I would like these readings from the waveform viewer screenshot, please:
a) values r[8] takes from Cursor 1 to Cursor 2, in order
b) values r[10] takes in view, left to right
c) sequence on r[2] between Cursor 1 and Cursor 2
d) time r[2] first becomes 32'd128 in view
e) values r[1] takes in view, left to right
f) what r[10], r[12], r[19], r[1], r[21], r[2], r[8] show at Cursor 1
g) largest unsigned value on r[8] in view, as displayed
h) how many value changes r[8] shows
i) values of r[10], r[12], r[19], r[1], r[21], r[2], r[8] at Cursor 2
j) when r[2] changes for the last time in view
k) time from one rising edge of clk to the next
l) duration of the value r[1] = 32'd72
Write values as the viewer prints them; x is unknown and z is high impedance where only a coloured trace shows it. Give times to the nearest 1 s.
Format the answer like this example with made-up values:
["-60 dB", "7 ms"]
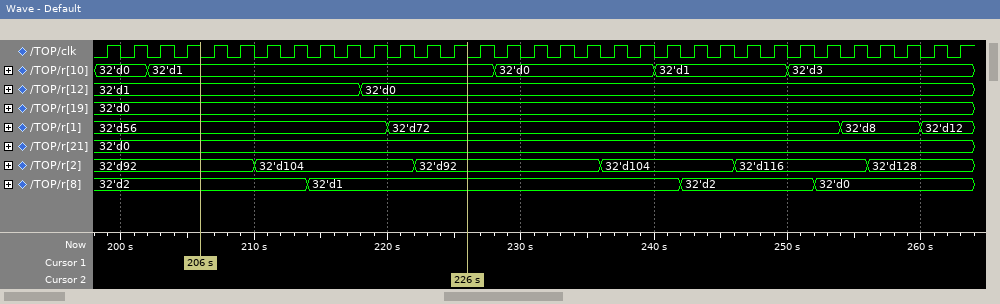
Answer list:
["32'd2, 32'd1", "32'd0, 32'd1, 32'd0, 32'd1, 32'd3", "32'd92, 32'd104, 32'd92", "256 s", "32'd56, 32'd72, 32'd8, 32'd12", "r[10]=32'd1, r[12]=32'd1, r[19]=32'd0, r[1]=32'd56, r[21]=32'd0, r[2]=32'd92, r[8]=32'd2", "32'd2", "3", "r[10]=32'd1, r[12]=32'd0, r[19]=32'd0, r[1]=32'd72, r[21]=32'd0, r[2]=32'd92, r[8]=32'd1", "256 s", "2 s", "34 s"]
